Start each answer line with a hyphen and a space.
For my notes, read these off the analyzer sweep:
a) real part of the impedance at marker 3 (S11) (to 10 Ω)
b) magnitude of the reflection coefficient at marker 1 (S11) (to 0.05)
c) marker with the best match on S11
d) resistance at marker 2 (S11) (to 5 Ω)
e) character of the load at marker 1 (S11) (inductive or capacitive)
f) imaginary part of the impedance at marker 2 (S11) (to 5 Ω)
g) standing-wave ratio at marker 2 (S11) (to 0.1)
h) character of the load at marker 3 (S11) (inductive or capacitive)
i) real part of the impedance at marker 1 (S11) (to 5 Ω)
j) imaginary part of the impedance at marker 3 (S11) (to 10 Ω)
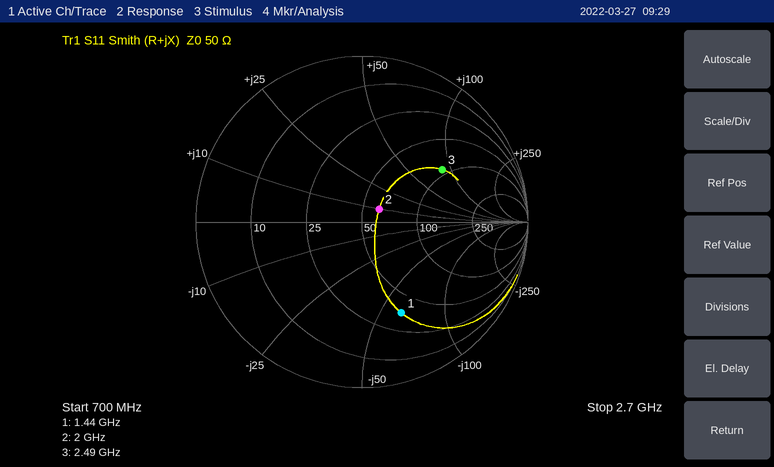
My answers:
- 90 Ω
- 0.60
- marker 2
- 60 Ω
- capacitive
- +10 Ω
- 1.3
- inductive
- 35 Ω
- +90 Ω
